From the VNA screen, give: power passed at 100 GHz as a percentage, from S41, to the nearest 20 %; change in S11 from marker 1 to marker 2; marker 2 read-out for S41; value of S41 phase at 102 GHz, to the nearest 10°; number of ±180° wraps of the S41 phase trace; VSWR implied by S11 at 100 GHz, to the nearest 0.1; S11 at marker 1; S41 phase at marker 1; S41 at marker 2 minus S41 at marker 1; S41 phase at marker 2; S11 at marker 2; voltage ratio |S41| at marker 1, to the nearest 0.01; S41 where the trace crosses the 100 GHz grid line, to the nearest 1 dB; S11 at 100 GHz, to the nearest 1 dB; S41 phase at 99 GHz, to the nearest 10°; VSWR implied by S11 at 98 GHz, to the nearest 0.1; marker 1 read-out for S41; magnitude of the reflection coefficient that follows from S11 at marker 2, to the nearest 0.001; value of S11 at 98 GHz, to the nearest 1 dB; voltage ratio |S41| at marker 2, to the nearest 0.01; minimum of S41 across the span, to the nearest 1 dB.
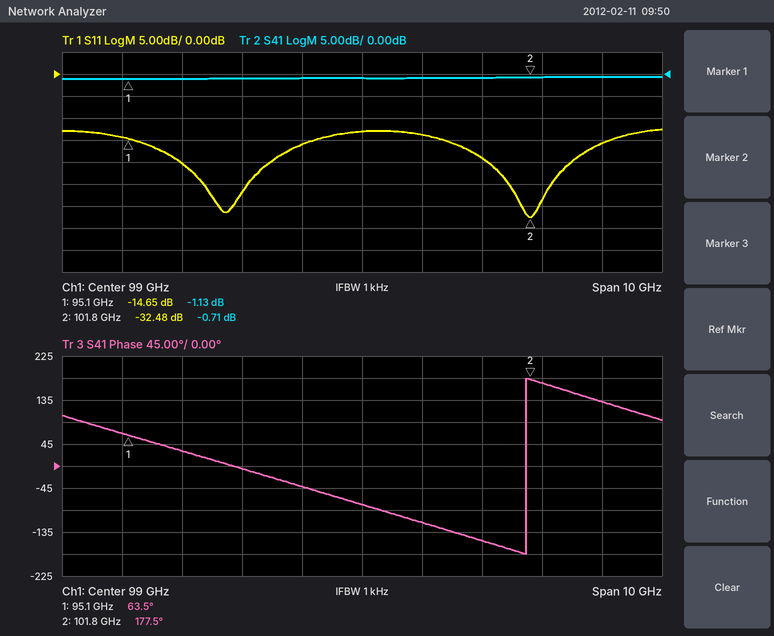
80 %
-17.83 dB
-0.71 dB
170°
1
1.5
-14.65 dB
63.5°
0.42 dB
177.5°
-32.48 dB
0.88
-1 dB
-14 dB
-80°
1.4
-1.13 dB
0.024
-16 dB
0.92
-1 dB
